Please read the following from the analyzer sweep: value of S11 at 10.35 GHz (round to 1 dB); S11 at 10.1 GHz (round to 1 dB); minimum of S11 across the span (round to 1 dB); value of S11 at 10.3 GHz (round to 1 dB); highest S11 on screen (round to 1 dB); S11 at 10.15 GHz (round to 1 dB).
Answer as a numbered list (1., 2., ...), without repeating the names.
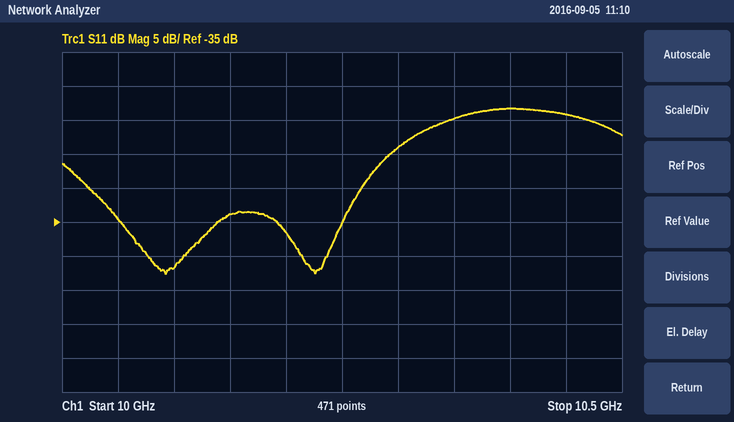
1. -20 dB
2. -42 dB
3. -43 dB
4. -24 dB
5. -18 dB
6. -34 dB
